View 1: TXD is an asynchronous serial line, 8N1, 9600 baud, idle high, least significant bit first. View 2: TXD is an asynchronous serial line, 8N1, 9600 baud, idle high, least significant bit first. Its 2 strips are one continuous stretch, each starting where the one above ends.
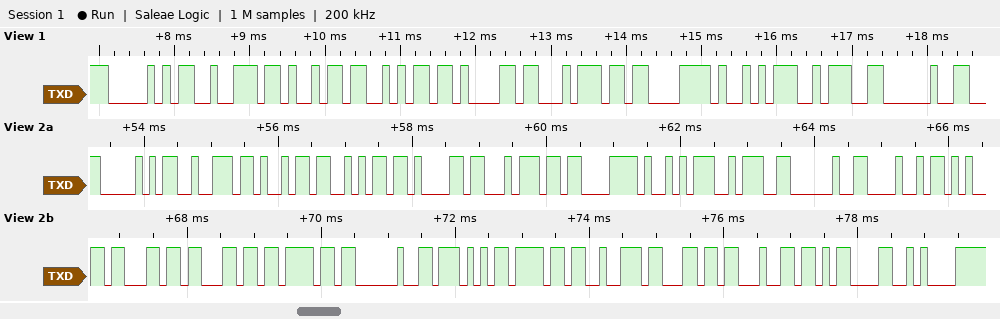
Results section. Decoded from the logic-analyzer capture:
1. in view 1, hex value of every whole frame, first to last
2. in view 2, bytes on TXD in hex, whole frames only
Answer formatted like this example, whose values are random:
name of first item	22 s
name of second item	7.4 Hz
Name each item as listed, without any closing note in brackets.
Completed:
in view 1, hex value of every whole frame, first to last	50 72 69 6A 61 74 C3 A9 3A 20
in view 2, bytes on TXD in hex, whole frames only	50 72 69 6A 61 74 C3 A9 3A 20 48 65 6C 6C 6F 20 57 6F 72 6C 64 0D 0A
